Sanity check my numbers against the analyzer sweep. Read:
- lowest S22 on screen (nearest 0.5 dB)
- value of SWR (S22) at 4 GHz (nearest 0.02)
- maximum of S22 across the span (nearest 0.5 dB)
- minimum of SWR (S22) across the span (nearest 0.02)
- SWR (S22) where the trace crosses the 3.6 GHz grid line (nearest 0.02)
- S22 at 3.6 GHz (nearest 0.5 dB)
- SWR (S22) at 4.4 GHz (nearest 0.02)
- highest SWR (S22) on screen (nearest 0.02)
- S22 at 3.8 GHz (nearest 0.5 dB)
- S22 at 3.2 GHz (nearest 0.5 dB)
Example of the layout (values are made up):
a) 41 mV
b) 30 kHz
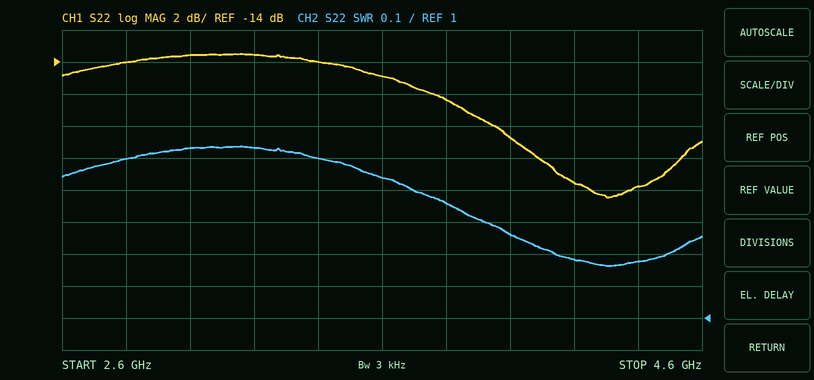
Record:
a) -22.5 dB
b) 1.26
c) -13.5 dB
d) 1.16
e) 1.44
f) -15.0 dB
g) 1.18
h) 1.54
i) -16.5 dB
j) -13.5 dB
